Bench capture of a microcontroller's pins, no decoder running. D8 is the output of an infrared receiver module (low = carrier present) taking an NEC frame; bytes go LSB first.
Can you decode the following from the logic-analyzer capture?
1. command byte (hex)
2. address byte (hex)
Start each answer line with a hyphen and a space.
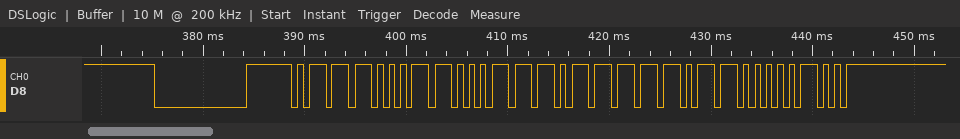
- 0xDF
- 0x8E
